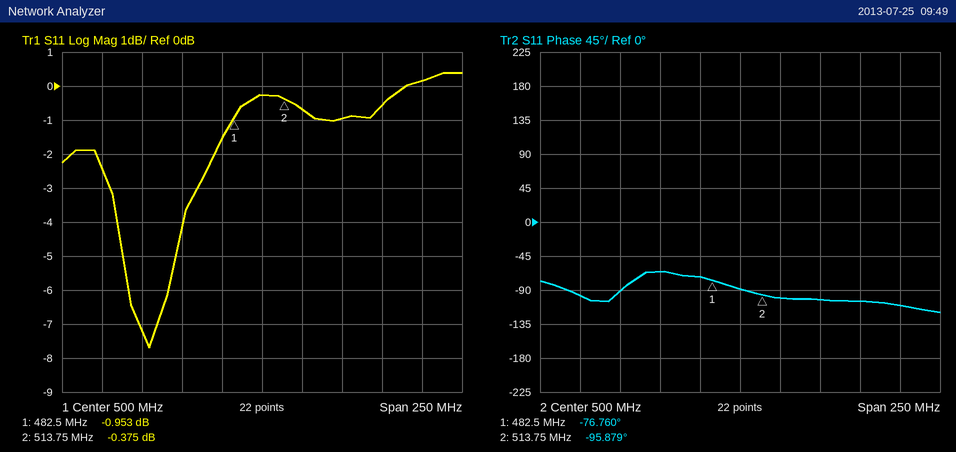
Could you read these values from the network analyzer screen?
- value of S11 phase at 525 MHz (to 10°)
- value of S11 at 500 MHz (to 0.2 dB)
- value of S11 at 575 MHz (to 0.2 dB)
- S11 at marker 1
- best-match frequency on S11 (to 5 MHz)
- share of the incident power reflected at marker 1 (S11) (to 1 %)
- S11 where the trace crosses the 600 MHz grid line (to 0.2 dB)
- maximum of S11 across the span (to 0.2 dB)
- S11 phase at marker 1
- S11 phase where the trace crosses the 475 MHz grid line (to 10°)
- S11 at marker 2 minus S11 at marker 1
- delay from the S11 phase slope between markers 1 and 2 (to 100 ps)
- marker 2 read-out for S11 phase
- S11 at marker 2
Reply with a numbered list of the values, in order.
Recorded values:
1. -100°
2. -0.2 dB
3. -0.6 dB
4. -0.953 dB
5. 430 MHz
6. 80 %
7. 0.2 dB
8. 0.4 dB
9. -76.760°
10. -70°
11. 0.578 dB
12. 1.7 ns
13. -95.879°
14. -0.375 dB
